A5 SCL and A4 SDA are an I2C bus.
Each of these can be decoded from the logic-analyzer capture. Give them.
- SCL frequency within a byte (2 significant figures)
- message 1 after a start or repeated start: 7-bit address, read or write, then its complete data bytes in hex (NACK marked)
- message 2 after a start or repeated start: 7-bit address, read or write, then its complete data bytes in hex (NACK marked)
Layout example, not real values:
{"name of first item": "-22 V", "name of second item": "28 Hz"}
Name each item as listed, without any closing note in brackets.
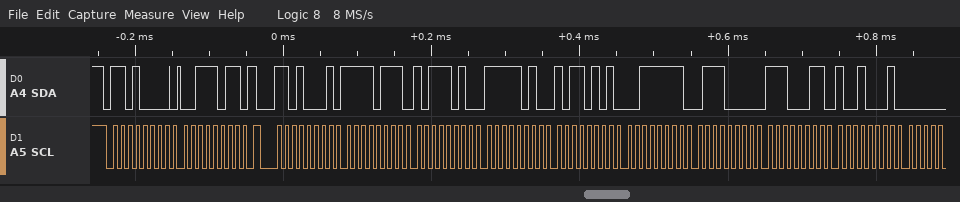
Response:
{"SCL frequency within a byte": "100 kHz", "message 1 after a start or repeated start: 7-bit address, read or write, then its complete data bytes in hex": "0x68 write: 3B", "message 2 after a start or repeated start: 7-bit address, read or write, then its complete data bytes in hex": "0x68 read: F7 BA FA B5 3F 70 E3 91"}
